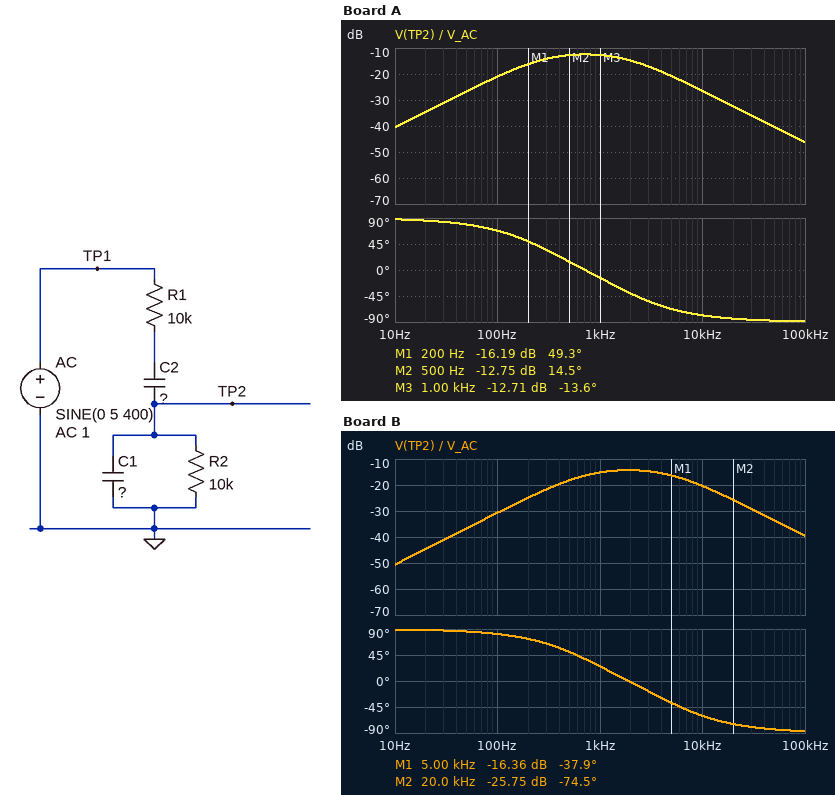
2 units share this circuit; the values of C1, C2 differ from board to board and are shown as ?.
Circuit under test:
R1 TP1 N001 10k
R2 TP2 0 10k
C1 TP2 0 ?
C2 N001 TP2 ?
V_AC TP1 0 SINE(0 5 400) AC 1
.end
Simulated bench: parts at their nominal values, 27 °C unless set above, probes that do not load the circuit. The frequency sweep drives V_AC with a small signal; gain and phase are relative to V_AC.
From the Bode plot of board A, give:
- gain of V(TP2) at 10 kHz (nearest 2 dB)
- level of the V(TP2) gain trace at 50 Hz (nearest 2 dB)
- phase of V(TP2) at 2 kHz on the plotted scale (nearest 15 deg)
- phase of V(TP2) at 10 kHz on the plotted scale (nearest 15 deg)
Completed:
-26 dB
-26 dB
-45 deg
-75 deg
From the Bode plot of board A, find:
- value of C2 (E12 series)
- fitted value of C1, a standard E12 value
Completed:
15 nF
33 nF
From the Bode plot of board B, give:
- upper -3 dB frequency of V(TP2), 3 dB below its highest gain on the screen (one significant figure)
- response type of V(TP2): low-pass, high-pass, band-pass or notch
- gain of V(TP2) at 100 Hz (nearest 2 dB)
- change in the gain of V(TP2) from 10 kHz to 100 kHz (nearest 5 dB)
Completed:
6 kHz
band-pass
-30 dB
-20 dB
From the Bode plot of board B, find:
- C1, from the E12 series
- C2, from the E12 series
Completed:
15 nF
4.7 nF
